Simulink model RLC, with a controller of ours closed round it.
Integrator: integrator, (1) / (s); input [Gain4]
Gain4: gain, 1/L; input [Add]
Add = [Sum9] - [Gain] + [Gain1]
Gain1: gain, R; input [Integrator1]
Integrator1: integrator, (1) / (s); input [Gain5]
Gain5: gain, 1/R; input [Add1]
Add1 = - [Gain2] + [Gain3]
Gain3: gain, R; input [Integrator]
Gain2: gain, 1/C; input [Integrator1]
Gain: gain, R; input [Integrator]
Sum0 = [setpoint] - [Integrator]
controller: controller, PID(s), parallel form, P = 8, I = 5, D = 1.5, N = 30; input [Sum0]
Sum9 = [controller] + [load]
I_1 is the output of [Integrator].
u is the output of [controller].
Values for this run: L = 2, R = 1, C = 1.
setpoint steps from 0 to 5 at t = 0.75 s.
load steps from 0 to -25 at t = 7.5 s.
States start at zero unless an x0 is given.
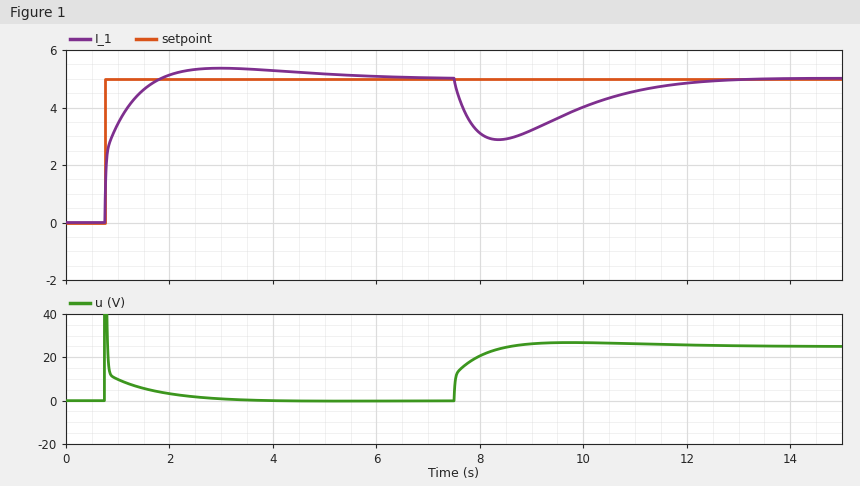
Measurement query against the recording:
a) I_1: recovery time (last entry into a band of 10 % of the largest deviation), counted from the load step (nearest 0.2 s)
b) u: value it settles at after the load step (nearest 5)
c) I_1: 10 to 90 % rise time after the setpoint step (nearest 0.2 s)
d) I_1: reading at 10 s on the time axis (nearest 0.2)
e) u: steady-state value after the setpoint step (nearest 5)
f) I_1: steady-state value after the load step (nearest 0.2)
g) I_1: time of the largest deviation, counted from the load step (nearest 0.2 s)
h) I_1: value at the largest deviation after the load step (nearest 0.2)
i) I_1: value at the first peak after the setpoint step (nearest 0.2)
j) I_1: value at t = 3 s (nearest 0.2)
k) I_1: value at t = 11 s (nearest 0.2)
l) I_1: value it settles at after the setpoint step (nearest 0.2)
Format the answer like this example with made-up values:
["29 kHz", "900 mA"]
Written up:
["4.2 s", "25", "0.6 s", "4.0", "0", "5.0", "0.8 s", "2.8", "5.4", "5.4", "4.6", "5.0"]
